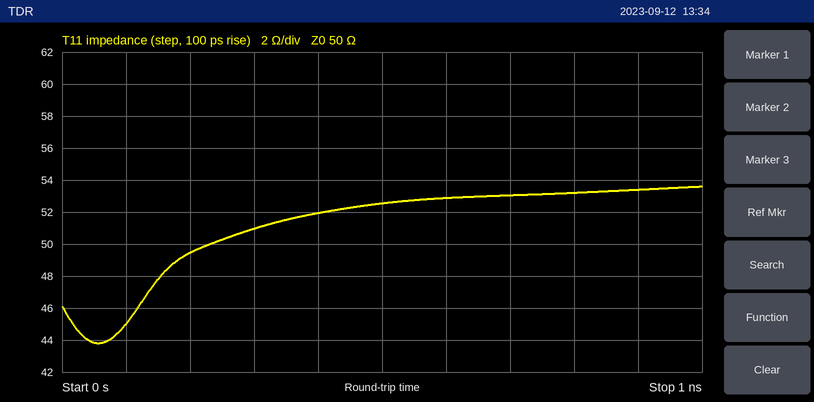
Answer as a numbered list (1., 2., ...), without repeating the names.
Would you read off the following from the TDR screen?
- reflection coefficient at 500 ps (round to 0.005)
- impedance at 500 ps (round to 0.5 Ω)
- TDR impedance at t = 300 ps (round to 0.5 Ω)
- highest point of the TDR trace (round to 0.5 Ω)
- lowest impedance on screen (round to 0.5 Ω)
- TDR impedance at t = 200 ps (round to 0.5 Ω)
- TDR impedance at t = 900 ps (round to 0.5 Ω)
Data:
1. +0.025
2. 52.5 Ω
3. 51.0 Ω
4. 53.5 Ω
5. 44.0 Ω
6. 49.5 Ω
7. 53.5 Ω
